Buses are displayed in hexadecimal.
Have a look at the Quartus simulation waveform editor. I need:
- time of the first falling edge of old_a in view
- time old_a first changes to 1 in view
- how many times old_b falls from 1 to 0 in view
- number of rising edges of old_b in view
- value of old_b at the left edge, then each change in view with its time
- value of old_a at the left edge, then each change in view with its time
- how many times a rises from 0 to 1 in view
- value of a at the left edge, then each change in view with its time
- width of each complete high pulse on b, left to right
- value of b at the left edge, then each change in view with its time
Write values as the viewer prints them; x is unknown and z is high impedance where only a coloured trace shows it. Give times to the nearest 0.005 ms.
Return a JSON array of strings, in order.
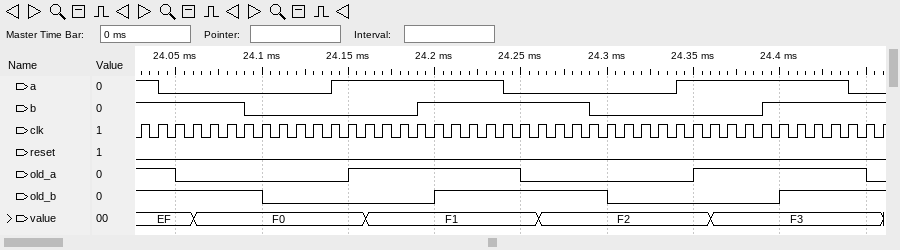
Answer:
["24.05 ms", "24.15 ms", "2", "2", "1, 0 at 24.1 ms, 1 at 24.2 ms, 0 at 24.3 ms, 1 at 24.4 ms", "1, 0 at 24.05 ms, 1 at 24.15 ms, 0 at 24.25 ms, 1 at 24.35 ms, 0 at 24.45 ms", "2", "1, 0 at 24.04 ms, 1 at 24.14 ms, 0 at 24.24 ms, 1 at 24.34 ms, 0 at 24.44 ms", "0.1 ms", "1, 0 at 24.09 ms, 1 at 24.19 ms, 0 at 24.29 ms, 1 at 24.39 ms"]
